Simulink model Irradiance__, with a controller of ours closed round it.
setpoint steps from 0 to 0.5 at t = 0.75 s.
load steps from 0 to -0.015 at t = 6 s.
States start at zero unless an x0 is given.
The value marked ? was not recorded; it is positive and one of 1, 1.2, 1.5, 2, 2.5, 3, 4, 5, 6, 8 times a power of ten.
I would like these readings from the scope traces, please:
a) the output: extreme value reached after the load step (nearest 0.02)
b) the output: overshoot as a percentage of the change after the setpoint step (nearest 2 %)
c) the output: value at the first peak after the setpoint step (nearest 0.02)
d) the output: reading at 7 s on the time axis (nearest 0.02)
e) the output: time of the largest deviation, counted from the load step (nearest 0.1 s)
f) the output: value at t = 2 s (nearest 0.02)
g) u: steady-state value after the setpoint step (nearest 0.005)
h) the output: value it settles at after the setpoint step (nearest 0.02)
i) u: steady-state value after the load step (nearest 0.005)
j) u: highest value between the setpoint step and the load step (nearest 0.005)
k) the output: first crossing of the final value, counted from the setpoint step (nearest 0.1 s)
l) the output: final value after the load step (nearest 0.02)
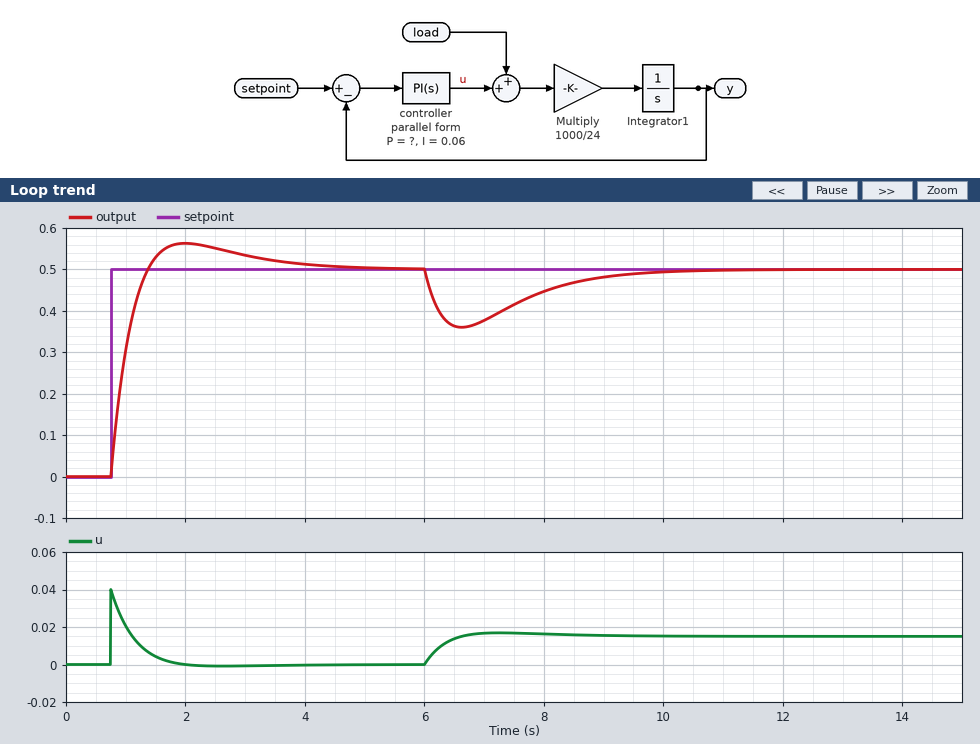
0.36
12 %
0.56
0.38
0.6 s
0.56
0.000
0.50
0.015
0.040
0.6 s
0.50
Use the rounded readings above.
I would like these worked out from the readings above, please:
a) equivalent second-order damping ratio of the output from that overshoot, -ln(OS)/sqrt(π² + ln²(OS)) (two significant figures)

0.56
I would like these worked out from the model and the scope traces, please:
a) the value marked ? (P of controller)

0.08
